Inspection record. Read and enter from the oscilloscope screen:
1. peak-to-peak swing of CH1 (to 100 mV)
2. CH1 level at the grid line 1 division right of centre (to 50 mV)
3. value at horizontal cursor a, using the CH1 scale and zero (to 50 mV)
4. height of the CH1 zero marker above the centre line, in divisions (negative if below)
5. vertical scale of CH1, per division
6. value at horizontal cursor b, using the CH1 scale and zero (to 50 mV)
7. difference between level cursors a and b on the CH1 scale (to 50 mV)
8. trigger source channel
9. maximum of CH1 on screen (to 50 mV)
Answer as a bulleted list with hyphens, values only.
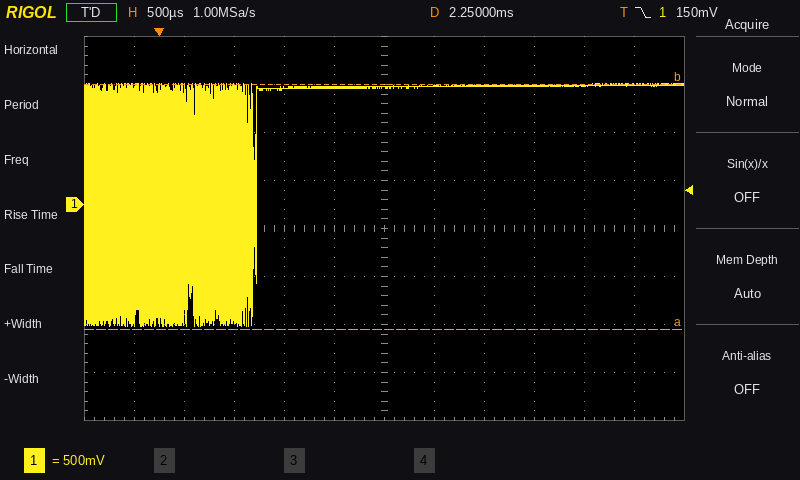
- 2.50 V
- 1.25 V
- -1.30 V
- +0.5 div
- 500 mV
- 1.25 V
- 2.55 V
- CH1
- 1.25 V
